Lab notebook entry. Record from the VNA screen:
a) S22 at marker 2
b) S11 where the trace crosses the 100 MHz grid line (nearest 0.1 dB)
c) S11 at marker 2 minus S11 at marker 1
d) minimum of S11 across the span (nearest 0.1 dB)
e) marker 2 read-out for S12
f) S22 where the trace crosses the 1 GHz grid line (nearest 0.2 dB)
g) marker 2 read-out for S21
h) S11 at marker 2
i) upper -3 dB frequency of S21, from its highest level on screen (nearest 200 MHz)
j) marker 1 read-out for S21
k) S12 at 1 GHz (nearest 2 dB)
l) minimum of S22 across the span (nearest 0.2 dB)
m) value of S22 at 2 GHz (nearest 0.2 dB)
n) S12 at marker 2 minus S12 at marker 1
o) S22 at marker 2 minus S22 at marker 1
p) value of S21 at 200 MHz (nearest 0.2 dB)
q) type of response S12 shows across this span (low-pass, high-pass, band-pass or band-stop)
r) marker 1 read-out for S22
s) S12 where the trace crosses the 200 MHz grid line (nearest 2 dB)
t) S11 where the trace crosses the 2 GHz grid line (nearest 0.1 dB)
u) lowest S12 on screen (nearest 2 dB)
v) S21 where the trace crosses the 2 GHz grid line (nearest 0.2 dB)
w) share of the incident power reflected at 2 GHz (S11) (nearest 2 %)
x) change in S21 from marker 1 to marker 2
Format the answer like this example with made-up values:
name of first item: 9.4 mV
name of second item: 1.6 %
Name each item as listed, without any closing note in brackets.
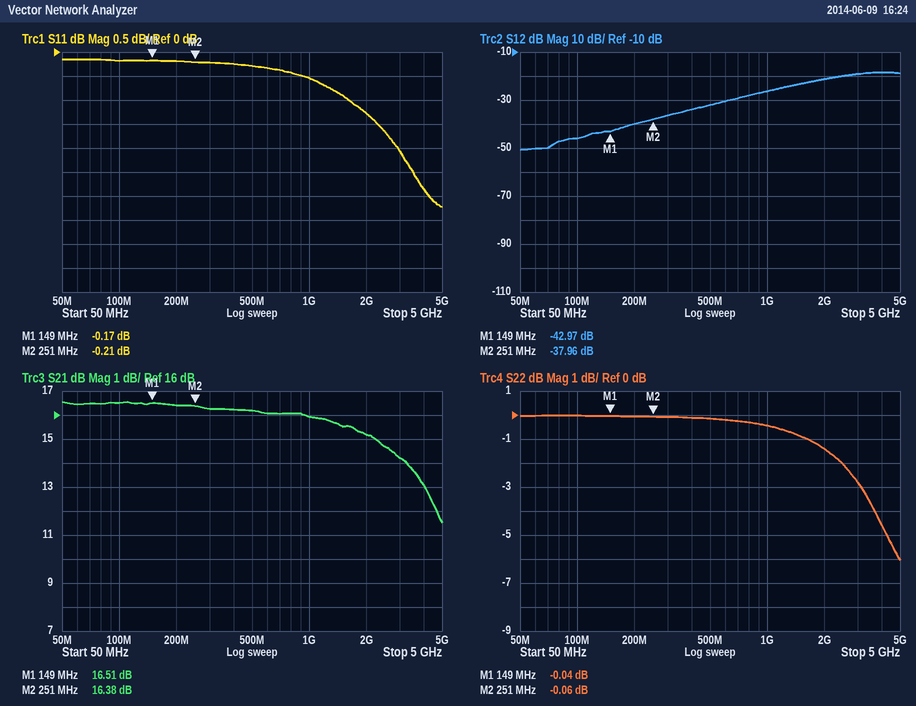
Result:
S22 at marker 2: -0.06 dB
S11 where the trace crosses the 100 MHz grid line: -0.2 dB
S11 at marker 2 minus S11 at marker 1: -0.04 dB
minimum of S11 across the span: -3.2 dB
marker 2 read-out for S12: -37.96 dB
S22 where the trace crosses the 1 GHz grid line: -0.4 dB
marker 2 read-out for S21: 16.38 dB
S11 at marker 2: -0.21 dB
upper -3 dB frequency of S21, from its highest level on screen: 3.6 GHz
marker 1 read-out for S21: 16.51 dB
S12 at 1 GHz: -26 dB
minimum of S22 across the span: -6.0 dB
value of S22 at 2 GHz: -1.4 dB
S12 at marker 2 minus S12 at marker 1: 5.01 dB
S22 at marker 2 minus S22 at marker 1: -0.02 dB
value of S21 at 200 MHz: 16.4 dB
type of response S12 shows across this span: high-pass
marker 1 read-out for S22: -0.04 dB
S12 where the trace crosses the 200 MHz grid line: -40 dB
S11 where the trace crosses the 2 GHz grid line: -1.3 dB
lowest S12 on screen: -50 dB
S21 where the trace crosses the 2 GHz grid line: 15.2 dB
share of the incident power reflected at 2 GHz (S11): 74 %
change in S21 from marker 1 to marker 2: -0.13 dB
